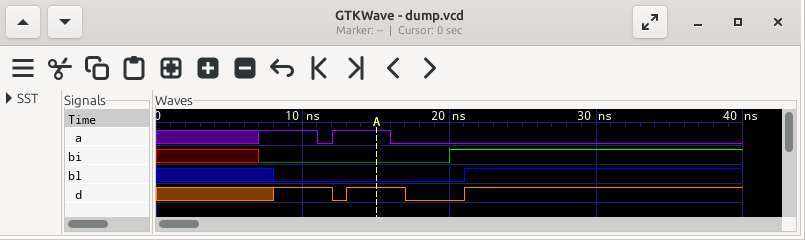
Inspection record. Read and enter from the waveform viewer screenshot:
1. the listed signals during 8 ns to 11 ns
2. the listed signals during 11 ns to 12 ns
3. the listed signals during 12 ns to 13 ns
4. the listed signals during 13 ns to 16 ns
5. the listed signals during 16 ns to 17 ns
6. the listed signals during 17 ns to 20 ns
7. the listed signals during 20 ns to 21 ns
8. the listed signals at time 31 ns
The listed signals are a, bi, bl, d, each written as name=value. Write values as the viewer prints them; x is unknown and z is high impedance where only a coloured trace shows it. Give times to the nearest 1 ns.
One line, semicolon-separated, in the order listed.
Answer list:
a=1, bi=0, bl=0, d=1; a=0, bi=0, bl=0, d=1; a=1, bi=0, bl=0, d=0; a=1, bi=0, bl=0, d=1; a=0, bi=0, bl=0, d=1; a=0, bi=0, bl=0, d=0; a=0, bi=1, bl=0, d=0; a=0, bi=1, bl=1, d=1
